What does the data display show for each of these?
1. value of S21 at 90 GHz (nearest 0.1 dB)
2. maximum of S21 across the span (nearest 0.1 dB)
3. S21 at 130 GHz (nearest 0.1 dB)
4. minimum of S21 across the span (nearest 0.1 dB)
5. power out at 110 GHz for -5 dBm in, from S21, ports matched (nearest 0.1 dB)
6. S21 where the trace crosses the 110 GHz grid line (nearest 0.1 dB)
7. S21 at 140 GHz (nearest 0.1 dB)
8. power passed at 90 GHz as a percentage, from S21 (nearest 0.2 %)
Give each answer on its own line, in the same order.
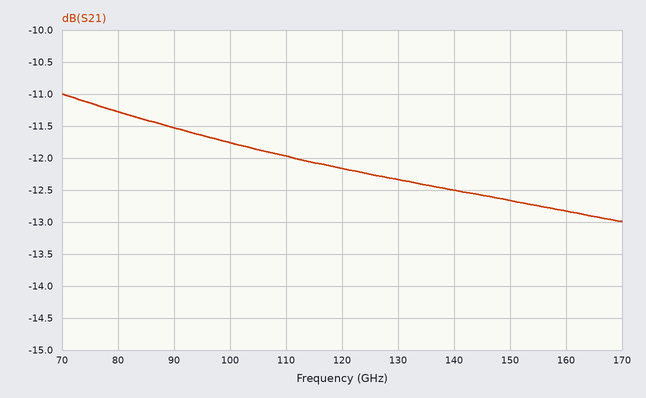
-11.5 dB
-11.0 dB
-12.3 dB
-13.0 dB
-17.0 dBm
-12.0 dB
-12.5 dB
7.0 %
